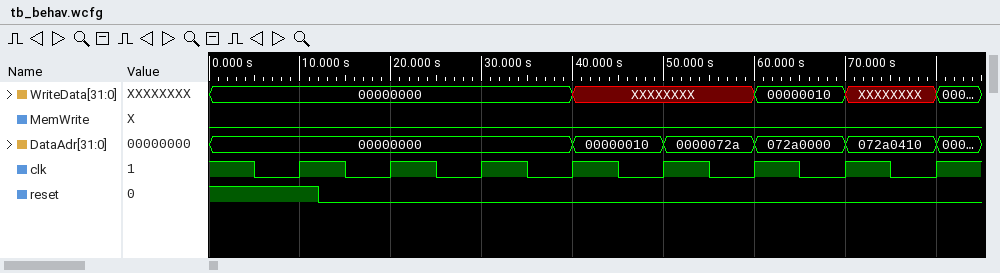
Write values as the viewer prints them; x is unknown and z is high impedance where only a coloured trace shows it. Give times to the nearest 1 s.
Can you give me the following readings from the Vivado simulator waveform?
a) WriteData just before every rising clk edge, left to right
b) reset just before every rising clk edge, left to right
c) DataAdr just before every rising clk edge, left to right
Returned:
00000000, 00000000, 00000000, 00000000, XXXXXXXX, XXXXXXXX, 00000010, XXXXXXXX
1 0 0 0 0 0 0 0
00000000, 00000000, 00000000, 00000000, 00000010, 0000072a, 072a0000, 072a0410
